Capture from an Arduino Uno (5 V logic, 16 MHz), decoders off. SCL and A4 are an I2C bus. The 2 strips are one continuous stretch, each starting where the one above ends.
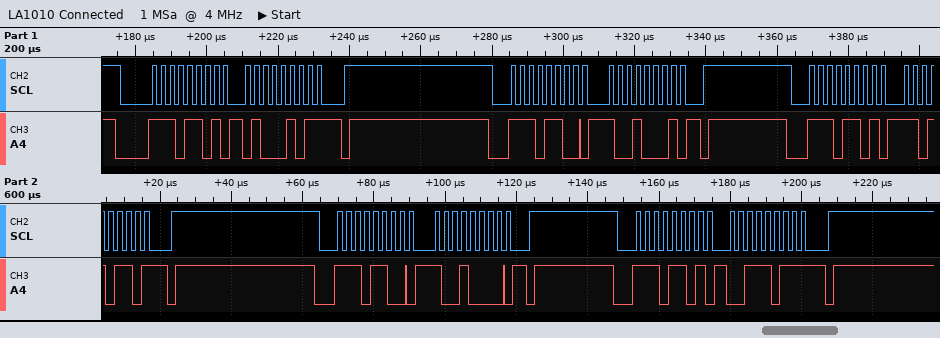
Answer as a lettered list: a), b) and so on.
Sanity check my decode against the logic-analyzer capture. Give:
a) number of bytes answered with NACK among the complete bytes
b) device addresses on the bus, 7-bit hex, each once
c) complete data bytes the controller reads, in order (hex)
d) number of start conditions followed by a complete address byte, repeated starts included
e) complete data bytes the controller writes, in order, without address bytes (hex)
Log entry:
a) 3
b) 0x76
c) 45 D6 3B
d) 5
e) 91 90
